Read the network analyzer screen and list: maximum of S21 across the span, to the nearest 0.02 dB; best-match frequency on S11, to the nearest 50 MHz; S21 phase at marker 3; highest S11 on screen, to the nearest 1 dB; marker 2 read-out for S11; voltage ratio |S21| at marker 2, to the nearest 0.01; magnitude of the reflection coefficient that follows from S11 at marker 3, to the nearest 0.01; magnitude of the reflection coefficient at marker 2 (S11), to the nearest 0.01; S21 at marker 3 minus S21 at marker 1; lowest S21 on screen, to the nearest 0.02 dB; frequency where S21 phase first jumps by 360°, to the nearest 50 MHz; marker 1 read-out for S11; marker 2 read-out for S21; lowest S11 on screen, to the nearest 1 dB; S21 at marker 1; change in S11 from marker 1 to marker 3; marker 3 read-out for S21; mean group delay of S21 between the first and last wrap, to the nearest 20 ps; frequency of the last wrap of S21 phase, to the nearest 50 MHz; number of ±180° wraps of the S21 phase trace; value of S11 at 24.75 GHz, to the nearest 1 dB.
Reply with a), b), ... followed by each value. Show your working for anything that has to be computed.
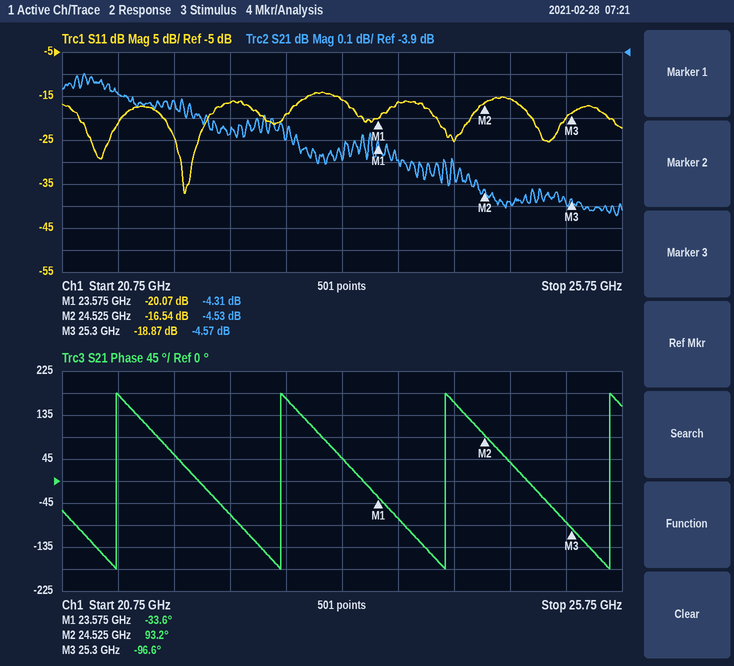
a) -4.00 dB
b) 21.85 GHz
c) -96.6°
d) -14 dB
e) -16.54 dB
f) 10^(-4.53/20) ≈ 0.59
g) 10^(-18.87/20) ≈ 0.11
h) 10^(-16.54/20) ≈ 0.15
i) -4.57 − (-4.31) = -0.26 dB
j) -4.64 dB
k) 21.25 GHz
l) -20.07 dB
m) -4.53 dB
n) -37 dB
o) -4.31 dB
p) -18.87 − (-20.07) = 1.20 dB
q) -4.57 dB
r) 3 cycles / (25.65 GHz − 21.25 GHz) ≈ 682 ps, so 680 ps to the nearest 20 ps
s) 25.65 GHz
t) 4
u) -16 dB
